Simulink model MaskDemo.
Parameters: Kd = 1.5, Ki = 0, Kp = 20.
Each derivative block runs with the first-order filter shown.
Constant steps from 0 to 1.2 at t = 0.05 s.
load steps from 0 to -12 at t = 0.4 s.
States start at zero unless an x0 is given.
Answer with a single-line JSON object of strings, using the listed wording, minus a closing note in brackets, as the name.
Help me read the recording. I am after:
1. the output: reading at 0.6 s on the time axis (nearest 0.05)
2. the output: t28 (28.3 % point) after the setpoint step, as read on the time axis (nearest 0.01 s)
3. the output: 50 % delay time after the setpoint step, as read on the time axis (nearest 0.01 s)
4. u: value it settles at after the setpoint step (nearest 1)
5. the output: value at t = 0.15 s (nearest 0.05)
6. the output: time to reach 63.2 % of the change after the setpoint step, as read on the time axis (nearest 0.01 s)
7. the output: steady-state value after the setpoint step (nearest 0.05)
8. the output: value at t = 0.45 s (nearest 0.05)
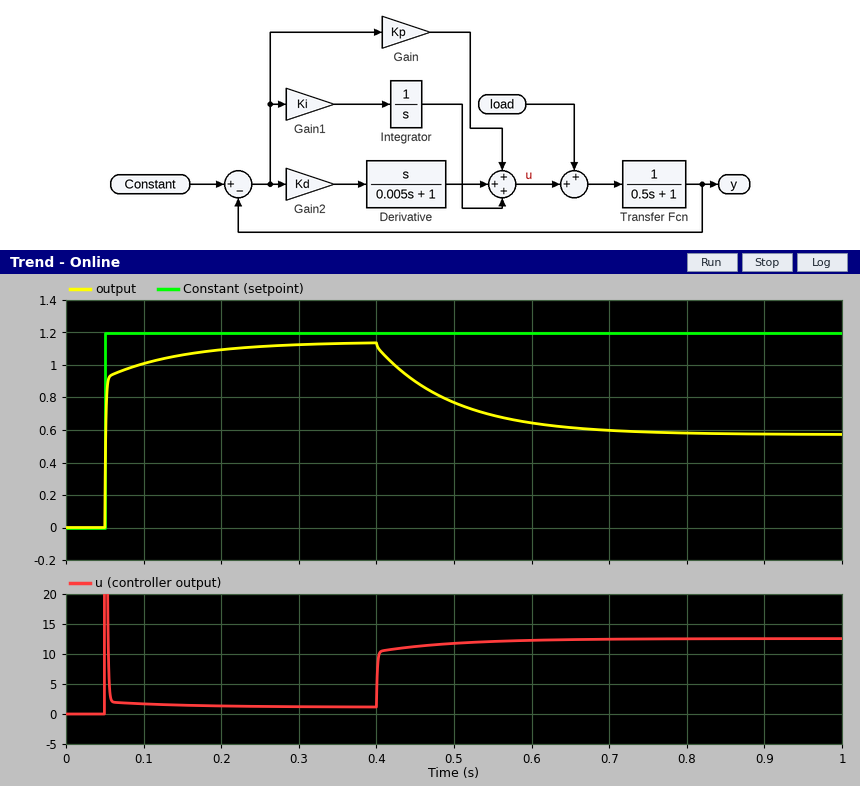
{"the output: reading at 0.6 s on the time axis": "0.65", "the output: t28 (28.3 % point) after the setpoint step, as read on the time axis": "0.05 s", "the output: 50 % delay time after the setpoint step, as read on the time axis": "0.05 s", "u: value it settles at after the setpoint step": "1", "the output: value at t = 0.15 s": "1.05", "the output: time to reach 63.2 % of the change after the setpoint step, as read on the time axis": "0.05 s", "the output: steady-state value after the setpoint step": "1.15", "the output: value at t = 0.45 s": "0.90"}
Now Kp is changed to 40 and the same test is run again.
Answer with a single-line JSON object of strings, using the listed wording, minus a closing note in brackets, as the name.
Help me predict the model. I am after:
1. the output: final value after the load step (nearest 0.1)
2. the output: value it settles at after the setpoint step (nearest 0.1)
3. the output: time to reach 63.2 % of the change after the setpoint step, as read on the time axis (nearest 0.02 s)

{"the output: final value after the load step": "0.9", "the output: value it settles at after the setpoint step": "1.2", "the output: time to reach 63.2 % of the change after the setpoint step, as read on the time axis": "0.06 s"}
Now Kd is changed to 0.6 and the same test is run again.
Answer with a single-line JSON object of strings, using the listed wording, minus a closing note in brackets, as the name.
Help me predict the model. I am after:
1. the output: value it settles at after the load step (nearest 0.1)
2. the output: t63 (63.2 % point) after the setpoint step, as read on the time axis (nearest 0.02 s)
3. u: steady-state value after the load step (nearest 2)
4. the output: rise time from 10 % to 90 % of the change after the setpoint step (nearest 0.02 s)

{"the output: value it settles at after the load step": "0.6", "the output: t63 (63.2 % point) after the setpoint step, as read on the time axis": "0.06 s", "u: steady-state value after the load step": "12", "the output: rise time from 10 % to 90 % of the change after the setpoint step": "0.08 s"}
